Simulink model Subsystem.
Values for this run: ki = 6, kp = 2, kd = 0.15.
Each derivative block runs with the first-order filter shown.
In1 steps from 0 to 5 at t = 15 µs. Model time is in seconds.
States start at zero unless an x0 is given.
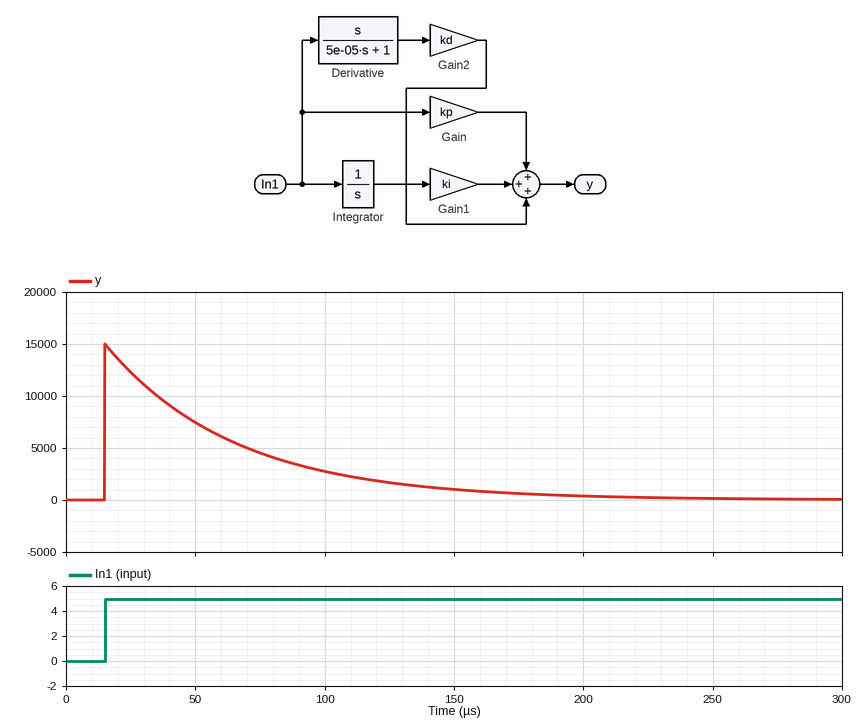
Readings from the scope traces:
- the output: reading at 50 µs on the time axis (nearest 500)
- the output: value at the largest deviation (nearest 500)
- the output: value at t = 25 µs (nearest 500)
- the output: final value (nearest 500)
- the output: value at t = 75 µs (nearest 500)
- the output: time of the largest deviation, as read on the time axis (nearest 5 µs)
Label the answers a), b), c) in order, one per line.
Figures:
a) 7500
b) 15000
c) 12500
d) 0
e) 4500
f) 15 µs
